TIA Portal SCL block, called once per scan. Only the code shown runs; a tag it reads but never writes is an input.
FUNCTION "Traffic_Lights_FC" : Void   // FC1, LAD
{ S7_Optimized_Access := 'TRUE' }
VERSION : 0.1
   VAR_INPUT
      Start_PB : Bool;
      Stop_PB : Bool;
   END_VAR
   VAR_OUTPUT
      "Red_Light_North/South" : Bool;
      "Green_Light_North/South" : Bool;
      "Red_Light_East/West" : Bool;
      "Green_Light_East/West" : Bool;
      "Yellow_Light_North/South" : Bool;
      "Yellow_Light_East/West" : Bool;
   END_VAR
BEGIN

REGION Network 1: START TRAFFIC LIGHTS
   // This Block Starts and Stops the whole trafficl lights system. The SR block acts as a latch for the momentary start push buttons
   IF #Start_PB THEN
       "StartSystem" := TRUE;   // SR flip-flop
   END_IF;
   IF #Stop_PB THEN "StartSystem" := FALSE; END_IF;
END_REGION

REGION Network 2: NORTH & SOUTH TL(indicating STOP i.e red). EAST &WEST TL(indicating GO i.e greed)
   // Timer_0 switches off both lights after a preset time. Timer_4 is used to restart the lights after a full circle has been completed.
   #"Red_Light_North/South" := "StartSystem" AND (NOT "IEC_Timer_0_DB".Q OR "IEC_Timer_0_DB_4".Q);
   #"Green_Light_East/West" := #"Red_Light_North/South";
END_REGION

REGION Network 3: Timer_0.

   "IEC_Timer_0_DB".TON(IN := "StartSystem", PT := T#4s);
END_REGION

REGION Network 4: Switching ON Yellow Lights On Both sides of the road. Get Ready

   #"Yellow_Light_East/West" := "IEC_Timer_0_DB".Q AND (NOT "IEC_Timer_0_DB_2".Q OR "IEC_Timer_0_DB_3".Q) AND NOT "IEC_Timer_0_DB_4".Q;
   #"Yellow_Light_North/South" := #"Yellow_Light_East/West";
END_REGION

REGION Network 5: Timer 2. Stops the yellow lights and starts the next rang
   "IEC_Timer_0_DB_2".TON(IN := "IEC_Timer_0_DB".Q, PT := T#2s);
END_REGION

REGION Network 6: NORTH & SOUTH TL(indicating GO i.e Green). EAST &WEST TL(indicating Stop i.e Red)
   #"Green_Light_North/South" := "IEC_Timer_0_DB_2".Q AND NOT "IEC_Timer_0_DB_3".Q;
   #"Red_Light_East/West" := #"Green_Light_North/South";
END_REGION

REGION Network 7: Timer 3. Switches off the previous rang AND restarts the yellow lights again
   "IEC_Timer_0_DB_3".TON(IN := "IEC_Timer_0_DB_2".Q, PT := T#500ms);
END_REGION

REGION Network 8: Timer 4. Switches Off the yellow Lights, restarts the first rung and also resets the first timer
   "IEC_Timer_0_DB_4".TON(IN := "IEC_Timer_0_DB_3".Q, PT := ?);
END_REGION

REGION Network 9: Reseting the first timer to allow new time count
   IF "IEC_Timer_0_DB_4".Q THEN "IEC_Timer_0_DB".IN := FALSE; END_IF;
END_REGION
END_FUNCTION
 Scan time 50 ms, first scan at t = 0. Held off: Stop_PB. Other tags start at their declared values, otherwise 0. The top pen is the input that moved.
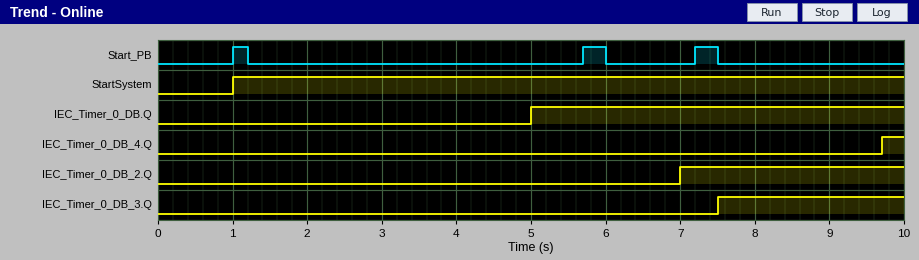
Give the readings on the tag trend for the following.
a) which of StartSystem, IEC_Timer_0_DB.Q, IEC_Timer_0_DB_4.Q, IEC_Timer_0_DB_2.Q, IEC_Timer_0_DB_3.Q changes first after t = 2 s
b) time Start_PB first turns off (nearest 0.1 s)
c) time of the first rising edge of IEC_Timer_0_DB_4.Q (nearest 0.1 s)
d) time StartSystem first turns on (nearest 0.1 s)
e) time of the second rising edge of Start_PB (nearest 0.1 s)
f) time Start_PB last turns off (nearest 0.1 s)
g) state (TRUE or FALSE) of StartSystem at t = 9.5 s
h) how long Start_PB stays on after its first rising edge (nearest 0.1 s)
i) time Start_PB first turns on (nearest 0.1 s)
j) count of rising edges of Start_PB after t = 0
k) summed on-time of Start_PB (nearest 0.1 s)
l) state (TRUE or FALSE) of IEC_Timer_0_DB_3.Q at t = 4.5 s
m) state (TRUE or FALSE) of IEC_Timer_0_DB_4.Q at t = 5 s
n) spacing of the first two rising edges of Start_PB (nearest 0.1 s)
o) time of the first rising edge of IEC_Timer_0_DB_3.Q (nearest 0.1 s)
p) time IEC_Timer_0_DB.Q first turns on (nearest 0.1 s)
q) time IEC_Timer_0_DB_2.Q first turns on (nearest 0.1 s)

IEC_Timer_0_DB.Q
1.2 s
9.7 s
1.0 s
5.7 s
7.5 s
TRUE
0.2 s
1.0 s
3
0.8 s
FALSE
FALSE
4.7 s
7.5 s
5.0 s
7.0 s
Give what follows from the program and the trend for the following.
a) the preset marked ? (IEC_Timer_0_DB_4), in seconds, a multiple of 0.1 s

2.2 s
